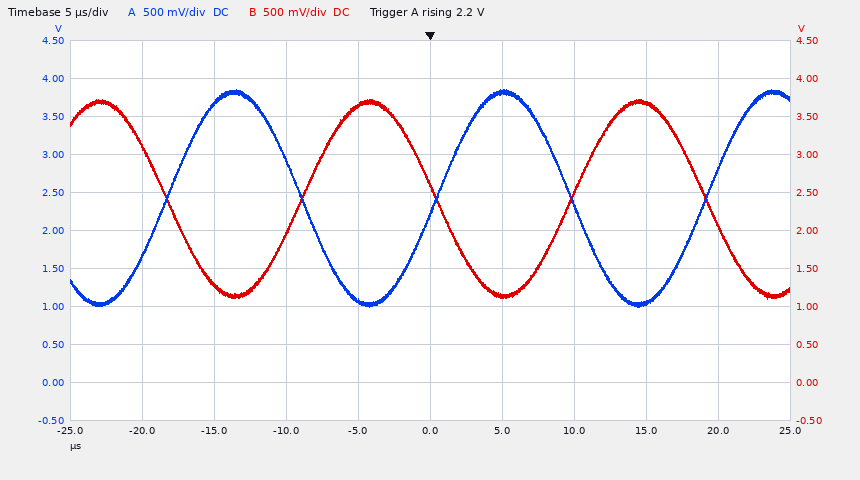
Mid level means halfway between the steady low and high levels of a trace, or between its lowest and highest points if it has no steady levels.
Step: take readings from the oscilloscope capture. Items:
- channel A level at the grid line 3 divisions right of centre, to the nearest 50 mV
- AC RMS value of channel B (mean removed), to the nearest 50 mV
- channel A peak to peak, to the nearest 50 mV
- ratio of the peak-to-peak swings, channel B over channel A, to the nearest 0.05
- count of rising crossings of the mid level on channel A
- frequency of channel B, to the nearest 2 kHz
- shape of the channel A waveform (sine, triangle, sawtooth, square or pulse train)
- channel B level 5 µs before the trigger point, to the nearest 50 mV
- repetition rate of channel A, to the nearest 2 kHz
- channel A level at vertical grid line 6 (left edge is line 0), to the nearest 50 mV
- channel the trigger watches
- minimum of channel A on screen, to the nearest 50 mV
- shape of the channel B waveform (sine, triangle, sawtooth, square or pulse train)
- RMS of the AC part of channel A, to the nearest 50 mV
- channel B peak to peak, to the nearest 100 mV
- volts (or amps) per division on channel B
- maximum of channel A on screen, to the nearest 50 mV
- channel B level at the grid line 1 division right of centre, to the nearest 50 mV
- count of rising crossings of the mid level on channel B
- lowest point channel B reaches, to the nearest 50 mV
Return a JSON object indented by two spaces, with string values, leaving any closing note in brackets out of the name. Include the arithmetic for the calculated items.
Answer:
{
  "channel A level at the grid line 3 divisions right of centre, to the nearest 50 mV": "1.05 V",
  "AC RMS value of channel B (mean removed), to the nearest 50 mV": "2.60 V / (2√2) ≈ 919 mV, so 900 mV to the nearest 50 mV",
  "channel A peak to peak, to the nearest 50 mV": "3.85 V − (1.00 V) = 2.85 V",
  "ratio of the peak-to-peak swings, channel B over channel A, to the nearest 0.05": "2.60 V / 2.85 V ≈ 0.912, so 0.90 to the nearest 0.05",
  "count of rising crossings of the mid level on channel A": "3",
  "frequency of channel B, to the nearest 2 kHz": "54 kHz",
  "shape of the channel A waveform": "sine",
  "channel B level 5 µs before the trigger point, to the nearest 50 mV": "3.65 V",
  "repetition rate of channel A, to the nearest 2 kHz": "54 kHz",
  "channel A level at vertical grid line 6 (left edge is line 0), to the nearest 50 mV": "3.80 V",
  "channel the trigger watches": "channel A",
  "minimum of channel A on screen, to the nearest 50 mV": "1.00 V",
  "shape of the channel B waveform": "sine",
  "RMS of the AC part of channel A, to the nearest 50 mV": "2.85 V / (2√2) ≈ 1.01 V, so 1.00 V to the nearest 50 mV",
  "channel B peak to peak, to the nearest 100 mV": "2.60 V",
  "volts (or amps) per division on channel B": "500 mV",
  "maximum of channel A on screen, to the nearest 50 mV": "3.85 V",
  "channel B level at the grid line 1 division right of centre, to the nearest 50 mV": "1.15 V",
  "count of rising crossings of the mid level on channel B": "2",
  "lowest point channel B reaches, to the nearest 50 mV": "1.10 V"
}
